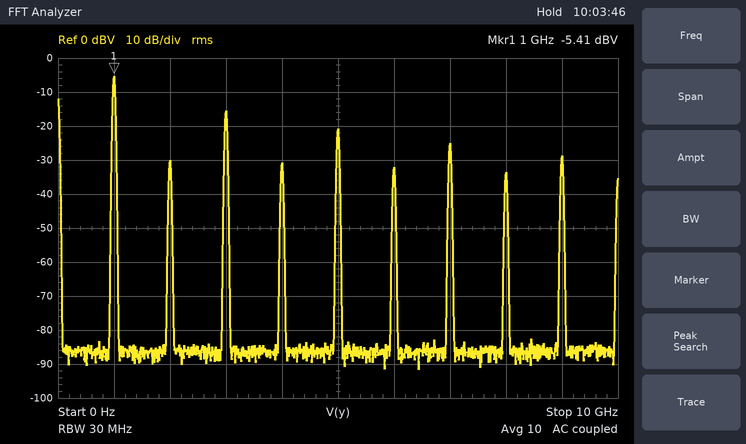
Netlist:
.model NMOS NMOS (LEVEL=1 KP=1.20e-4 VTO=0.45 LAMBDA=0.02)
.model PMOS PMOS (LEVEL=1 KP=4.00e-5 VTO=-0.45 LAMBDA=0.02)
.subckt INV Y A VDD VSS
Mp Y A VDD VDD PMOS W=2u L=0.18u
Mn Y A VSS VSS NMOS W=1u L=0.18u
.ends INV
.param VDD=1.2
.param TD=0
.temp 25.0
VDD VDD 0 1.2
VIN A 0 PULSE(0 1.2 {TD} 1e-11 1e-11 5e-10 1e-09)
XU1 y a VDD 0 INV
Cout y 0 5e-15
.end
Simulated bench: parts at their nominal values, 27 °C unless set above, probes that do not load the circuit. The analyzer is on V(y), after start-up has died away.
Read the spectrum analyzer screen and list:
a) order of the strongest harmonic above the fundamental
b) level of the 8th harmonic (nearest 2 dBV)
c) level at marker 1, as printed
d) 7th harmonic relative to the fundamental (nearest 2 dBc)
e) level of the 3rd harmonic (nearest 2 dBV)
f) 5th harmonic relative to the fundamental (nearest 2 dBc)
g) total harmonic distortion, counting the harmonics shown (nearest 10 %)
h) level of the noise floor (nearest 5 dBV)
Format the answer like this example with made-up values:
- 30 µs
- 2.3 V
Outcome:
- 3
- -34 dBV
- -5.41 dBV
- -20 dBc
- -16 dBV
- -16 dBc
- 40 %
- -85 dBV
